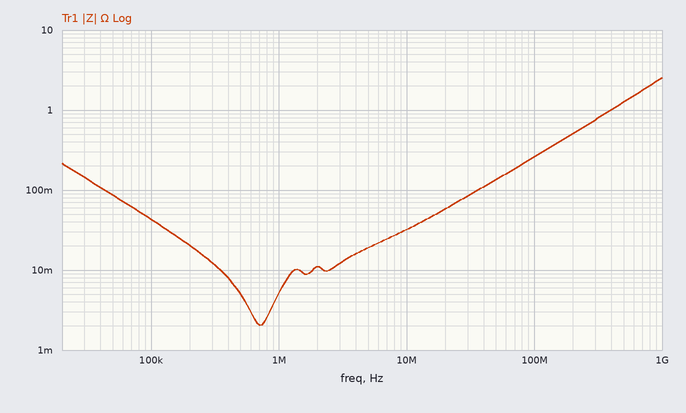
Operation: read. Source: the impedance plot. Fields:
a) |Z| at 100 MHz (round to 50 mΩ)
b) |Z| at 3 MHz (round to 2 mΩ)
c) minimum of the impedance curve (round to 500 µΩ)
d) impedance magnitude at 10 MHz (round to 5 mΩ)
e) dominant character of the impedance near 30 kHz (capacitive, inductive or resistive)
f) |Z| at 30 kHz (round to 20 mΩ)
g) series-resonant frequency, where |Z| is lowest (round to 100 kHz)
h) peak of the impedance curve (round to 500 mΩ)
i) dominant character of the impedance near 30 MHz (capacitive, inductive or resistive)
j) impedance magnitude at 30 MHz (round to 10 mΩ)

250 mΩ
12 mΩ
2.0 mΩ
30 mΩ
capacitive
140 mΩ
700 kHz
2.5 Ω
inductive
80 mΩ
